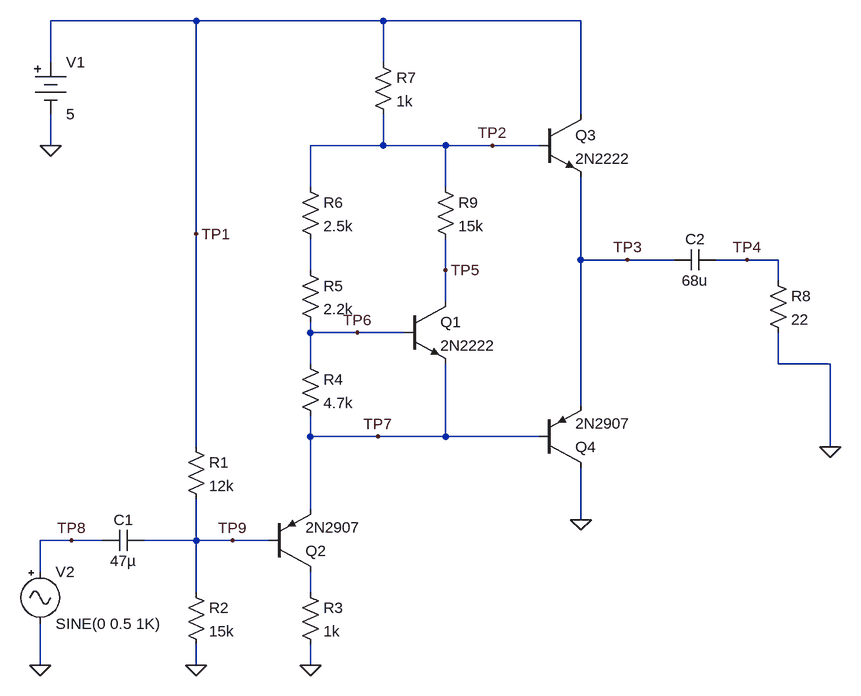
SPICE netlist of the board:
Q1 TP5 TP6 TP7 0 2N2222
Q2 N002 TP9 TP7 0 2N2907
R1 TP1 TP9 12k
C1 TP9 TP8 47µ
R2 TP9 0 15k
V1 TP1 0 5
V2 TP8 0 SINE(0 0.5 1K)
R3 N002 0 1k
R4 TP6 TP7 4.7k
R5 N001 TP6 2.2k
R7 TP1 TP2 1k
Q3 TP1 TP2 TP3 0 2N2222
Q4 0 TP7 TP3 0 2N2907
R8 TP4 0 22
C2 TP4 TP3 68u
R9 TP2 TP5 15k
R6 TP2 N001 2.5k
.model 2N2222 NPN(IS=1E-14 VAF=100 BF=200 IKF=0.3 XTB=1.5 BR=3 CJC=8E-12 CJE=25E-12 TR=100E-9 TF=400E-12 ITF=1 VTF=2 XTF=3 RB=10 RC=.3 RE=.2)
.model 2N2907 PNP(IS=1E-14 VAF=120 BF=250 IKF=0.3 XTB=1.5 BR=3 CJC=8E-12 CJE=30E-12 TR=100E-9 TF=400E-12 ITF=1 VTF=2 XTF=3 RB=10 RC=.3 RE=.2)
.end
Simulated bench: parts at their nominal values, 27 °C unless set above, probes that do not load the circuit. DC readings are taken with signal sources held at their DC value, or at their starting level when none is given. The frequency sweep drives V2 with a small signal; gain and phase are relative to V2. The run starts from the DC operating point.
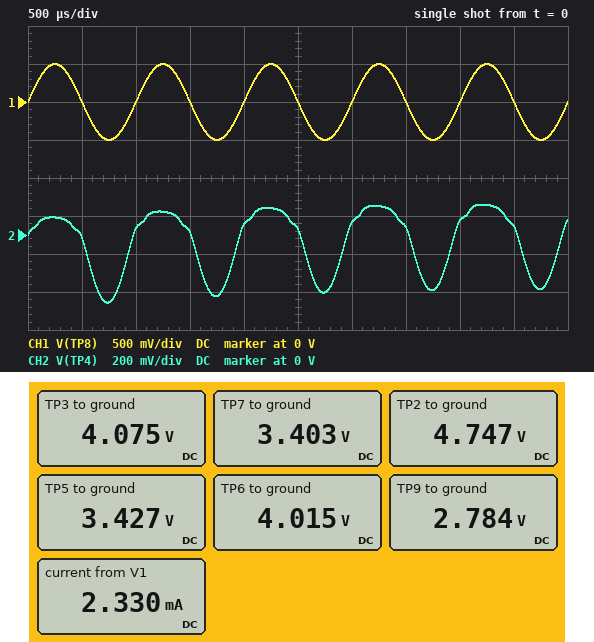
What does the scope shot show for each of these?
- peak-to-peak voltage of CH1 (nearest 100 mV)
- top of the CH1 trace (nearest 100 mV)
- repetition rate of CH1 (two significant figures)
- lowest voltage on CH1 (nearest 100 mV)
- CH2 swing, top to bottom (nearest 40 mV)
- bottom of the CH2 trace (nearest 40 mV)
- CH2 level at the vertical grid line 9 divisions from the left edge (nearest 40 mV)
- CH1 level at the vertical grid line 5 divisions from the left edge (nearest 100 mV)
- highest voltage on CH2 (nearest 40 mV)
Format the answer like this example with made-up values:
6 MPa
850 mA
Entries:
1.0 V
500 mV
1.0 kHz
-500 mV
520 mV
-360 mV
40 mV
0 V
160 mV
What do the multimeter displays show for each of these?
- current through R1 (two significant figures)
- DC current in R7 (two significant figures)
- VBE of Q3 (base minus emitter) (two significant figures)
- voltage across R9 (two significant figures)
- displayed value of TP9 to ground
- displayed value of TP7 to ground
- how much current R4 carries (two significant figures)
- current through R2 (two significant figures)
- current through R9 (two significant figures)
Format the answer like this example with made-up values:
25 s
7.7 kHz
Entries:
180 µA
250 µA
670 mV
1.3 V
2.784 V
3.403 V
130 µA
190 µA
88 µA
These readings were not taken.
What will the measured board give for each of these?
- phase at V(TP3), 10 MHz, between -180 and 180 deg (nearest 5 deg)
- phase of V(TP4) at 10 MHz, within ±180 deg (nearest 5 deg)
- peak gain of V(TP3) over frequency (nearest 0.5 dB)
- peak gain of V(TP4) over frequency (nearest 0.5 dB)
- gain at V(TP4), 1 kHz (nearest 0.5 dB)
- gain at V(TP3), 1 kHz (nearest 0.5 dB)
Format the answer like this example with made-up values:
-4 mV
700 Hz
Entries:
-5 deg
-5 deg
-4.0 dB
-6.0 dB
-6.5 dB
-6.5 dB
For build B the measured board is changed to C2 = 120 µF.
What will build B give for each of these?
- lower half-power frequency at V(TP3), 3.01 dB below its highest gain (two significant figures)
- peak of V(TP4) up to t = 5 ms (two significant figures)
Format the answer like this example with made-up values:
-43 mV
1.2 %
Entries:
500 mHz
150 mV
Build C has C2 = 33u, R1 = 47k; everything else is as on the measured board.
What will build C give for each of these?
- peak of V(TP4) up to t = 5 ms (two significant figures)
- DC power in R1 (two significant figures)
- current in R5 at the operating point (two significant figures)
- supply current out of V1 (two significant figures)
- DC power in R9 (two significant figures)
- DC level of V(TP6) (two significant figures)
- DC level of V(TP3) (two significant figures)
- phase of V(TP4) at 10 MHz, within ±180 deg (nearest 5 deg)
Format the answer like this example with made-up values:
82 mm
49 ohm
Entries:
440 mV
300 µW
220 µA
150 mA
180 µW
2.6 V
2.8 V
-5 deg
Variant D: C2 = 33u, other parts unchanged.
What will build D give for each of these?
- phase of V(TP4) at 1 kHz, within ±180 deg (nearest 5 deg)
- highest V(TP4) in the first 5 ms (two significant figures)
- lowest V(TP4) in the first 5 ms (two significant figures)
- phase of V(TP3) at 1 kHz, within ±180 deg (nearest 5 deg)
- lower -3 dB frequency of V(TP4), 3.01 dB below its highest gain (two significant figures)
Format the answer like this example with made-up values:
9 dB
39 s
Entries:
10 deg
170 mV
-340 mV
-5 deg
190 Hz
